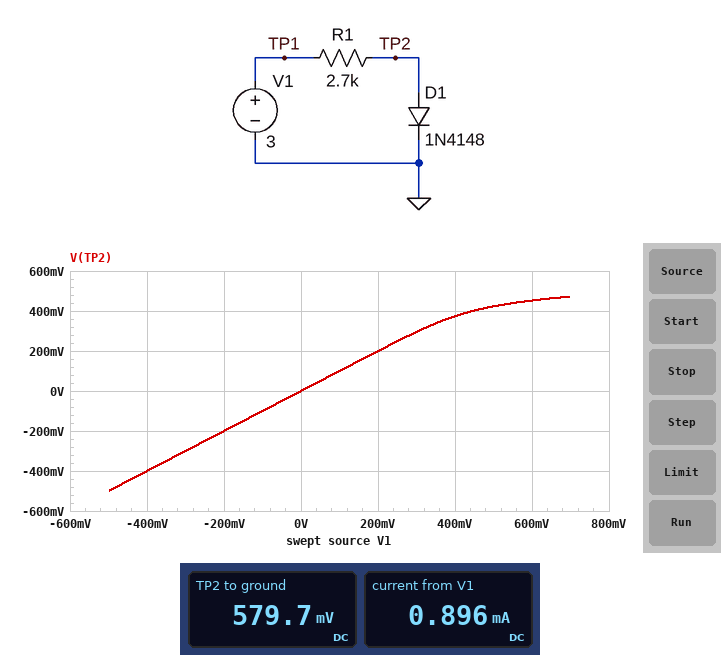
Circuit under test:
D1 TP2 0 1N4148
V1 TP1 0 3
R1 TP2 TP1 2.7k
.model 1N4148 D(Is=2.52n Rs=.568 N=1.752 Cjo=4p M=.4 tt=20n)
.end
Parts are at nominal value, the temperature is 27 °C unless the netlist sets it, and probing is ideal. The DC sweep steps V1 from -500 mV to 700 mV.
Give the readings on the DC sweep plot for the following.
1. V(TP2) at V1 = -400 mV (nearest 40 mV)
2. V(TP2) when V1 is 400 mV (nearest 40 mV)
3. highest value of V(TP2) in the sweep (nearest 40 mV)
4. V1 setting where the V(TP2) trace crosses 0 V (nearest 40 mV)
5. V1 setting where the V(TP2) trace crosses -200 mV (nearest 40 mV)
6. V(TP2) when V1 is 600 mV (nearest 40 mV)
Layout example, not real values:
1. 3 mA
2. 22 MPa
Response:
1. -400 mV
2. 360 mV
3. 480 mV
4. 0 V
5. -200 mV
6. 440 mV
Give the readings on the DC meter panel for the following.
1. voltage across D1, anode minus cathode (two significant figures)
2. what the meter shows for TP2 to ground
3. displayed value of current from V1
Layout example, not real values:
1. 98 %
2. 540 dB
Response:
1. 580 mV
2. 579.7 mV
3. 0.896 mA
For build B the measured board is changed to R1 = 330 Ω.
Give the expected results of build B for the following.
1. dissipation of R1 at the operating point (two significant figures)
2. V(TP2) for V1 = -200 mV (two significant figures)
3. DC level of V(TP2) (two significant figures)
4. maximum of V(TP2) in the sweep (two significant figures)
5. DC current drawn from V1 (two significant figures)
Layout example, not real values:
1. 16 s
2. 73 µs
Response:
1. 16 mW
2. -200 mV
3. 680 mV
4. 550 mV
5. 7.0 mA
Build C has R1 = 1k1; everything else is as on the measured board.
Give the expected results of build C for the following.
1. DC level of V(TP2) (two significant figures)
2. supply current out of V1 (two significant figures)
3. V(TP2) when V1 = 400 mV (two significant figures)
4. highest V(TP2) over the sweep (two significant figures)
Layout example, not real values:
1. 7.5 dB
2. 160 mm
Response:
1. 620 mV
2. 2.2 mA
3. 390 mV
4. 510 mV
